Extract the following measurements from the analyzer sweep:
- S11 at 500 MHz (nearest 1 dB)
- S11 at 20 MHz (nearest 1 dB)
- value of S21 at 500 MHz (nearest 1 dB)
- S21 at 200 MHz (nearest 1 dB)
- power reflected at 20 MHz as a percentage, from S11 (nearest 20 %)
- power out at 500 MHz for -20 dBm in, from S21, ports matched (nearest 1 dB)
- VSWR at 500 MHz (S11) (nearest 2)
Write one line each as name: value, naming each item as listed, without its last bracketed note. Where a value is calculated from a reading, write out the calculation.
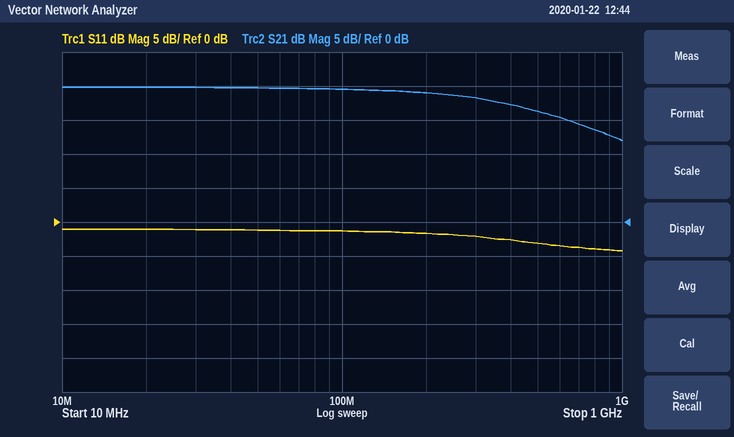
S11 at 500 MHz: -3 dB
S11 at 20 MHz: -1 dB
value of S21 at 500 MHz: 16 dB
S21 at 200 MHz: 19 dB
power reflected at 20 MHz as a percentage, from S11: 10^(-1/10) ≈ 79.4 %, so 80 % to the nearest 20 %
power out at 500 MHz for -20 dBm in, from S21, ports matched: -20 dBm + (16 dB) = -4 dBm
VSWR at 500 MHz (S11): |Γ| = 10^(-3/20) = 0.7079; VSWR = (1 + 0.7079)/(1 − 0.7079) ≈ 6
